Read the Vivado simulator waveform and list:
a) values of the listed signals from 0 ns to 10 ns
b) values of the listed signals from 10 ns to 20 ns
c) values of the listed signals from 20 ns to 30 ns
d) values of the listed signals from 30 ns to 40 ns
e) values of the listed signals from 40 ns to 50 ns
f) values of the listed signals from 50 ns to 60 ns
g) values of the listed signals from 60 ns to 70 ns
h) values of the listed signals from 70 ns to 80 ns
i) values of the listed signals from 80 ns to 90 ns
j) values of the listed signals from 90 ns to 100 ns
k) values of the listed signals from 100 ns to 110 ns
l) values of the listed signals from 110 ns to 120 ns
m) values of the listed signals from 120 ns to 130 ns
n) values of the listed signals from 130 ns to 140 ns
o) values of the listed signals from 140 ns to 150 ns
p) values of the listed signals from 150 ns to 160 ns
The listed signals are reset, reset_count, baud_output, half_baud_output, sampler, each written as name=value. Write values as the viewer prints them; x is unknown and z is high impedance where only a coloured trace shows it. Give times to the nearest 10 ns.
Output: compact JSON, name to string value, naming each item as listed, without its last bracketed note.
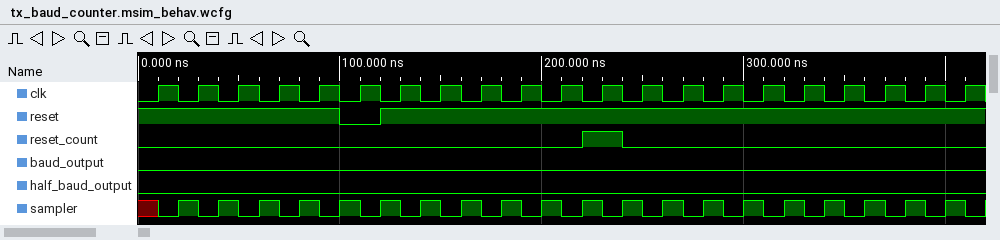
{"values of the listed signals from 0 ns to 10 ns": "reset=1, reset_count=0, baud_output=0, half_baud_output=0, sampler=x", "values of the listed signals from 10 ns to 20 ns": "reset=1, reset_count=0, baud_output=0, half_baud_output=0, sampler=0", "values of the listed signals from 20 ns to 30 ns": "reset=1, reset_count=0, baud_output=0, half_baud_output=0, sampler=1", "values of the listed signals from 30 ns to 40 ns": "reset=1, reset_count=0, baud_output=0, half_baud_output=0, sampler=0", "values of the listed signals from 40 ns to 50 ns": "reset=1, reset_count=0, baud_output=0, half_baud_output=0, sampler=1", "values of the listed signals from 50 ns to 60 ns": "reset=1, reset_count=0, baud_output=0, half_baud_output=0, sampler=0", "values of the listed signals from 60 ns to 70 ns": "reset=1, reset_count=0, baud_output=0, half_baud_output=0, sampler=1", "values of the listed signals from 70 ns to 80 ns": "reset=1, reset_count=0, baud_output=0, half_baud_output=0, sampler=0", "values of the listed signals from 80 ns to 90 ns": "reset=1, reset_count=0, baud_output=0, half_baud_output=0, sampler=1", "values of the listed signals from 90 ns to 100 ns": "reset=1, reset_count=0, baud_output=0, half_baud_output=0, sampler=0", "values of the listed signals from 100 ns to 110 ns": "reset=0, reset_count=0, baud_output=0, half_baud_output=0, sampler=1", "values of the listed signals from 110 ns to 120 ns": "reset=0, reset_count=0, baud_output=0, half_baud_output=0, sampler=0", "values of the listed signals from 120 ns to 130 ns": "reset=1, reset_count=0, baud_output=0, half_baud_output=0, sampler=1", "values of the listed signals from 130 ns to 140 ns": "reset=1, reset_count=0, baud_output=0, half_baud_output=0, sampler=0", "values of the listed signals from 140 ns to 150 ns": "reset=1, reset_count=0, baud_output=0, half_baud_output=0, sampler=1", "values of the listed signals from 150 ns to 160 ns": "reset=1, reset_count=0, baud_output=0, half_baud_output=0, sampler=0"}
